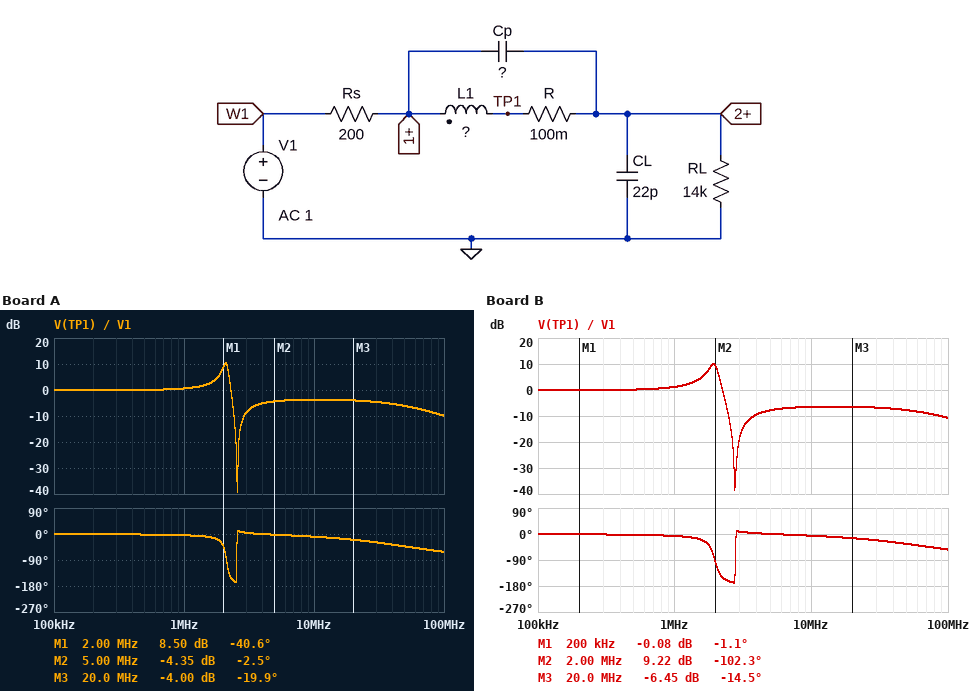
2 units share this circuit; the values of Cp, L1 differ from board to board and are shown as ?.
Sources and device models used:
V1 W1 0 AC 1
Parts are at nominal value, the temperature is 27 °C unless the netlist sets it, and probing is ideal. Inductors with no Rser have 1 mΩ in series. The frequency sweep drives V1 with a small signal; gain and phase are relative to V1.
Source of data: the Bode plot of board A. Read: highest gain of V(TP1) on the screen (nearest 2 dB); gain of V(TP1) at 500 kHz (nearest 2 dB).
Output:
10 dB
0 dB
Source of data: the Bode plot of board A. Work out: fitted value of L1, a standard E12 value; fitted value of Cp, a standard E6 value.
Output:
82 µH
47 pF
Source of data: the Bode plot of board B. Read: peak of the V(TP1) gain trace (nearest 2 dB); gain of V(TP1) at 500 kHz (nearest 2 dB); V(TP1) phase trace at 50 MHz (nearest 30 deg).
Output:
10 dB
0 dB
-30 deg
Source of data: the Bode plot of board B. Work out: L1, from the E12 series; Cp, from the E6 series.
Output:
150 µH
22 pF
